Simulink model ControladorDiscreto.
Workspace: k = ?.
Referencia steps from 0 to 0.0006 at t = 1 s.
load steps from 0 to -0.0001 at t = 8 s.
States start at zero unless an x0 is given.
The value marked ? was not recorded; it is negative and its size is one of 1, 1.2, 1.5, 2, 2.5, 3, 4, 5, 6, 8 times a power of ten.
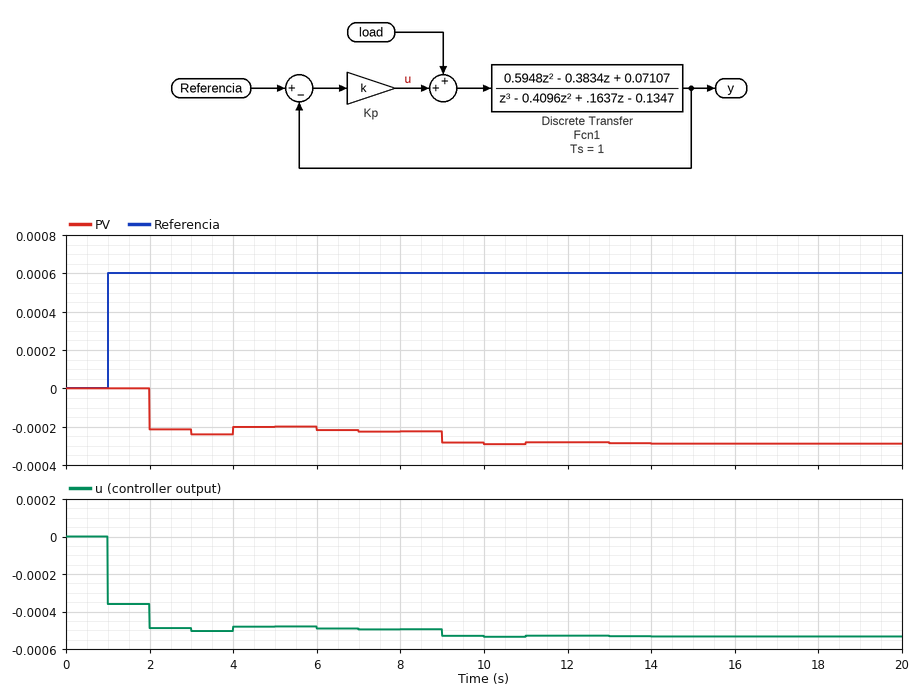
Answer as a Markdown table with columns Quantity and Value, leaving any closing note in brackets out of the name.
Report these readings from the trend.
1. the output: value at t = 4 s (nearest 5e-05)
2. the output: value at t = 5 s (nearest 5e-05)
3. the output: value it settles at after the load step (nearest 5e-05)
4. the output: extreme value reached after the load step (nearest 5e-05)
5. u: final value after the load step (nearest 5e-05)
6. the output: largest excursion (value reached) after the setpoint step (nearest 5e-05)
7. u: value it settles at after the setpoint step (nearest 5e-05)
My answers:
| Quantity | Value |
|---|---|
| the output: value at t = 4 s | -0.00020 |
| the output: value at t = 5 s | -0.00020 |
| the output: value it settles at after the load step | -0.00030 |
| the output: extreme value reached after the load step | -0.00030 |
| u: final value after the load step | -0.00055 |
| the output: largest excursion (value reached) after the setpoint step | -0.00025 |
| u: value it settles at after the setpoint step | -0.00050 |
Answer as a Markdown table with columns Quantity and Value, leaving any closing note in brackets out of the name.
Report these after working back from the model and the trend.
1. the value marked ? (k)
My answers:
| Quantity | Value |
|---|---|
| the value marked ? | -0.6 |
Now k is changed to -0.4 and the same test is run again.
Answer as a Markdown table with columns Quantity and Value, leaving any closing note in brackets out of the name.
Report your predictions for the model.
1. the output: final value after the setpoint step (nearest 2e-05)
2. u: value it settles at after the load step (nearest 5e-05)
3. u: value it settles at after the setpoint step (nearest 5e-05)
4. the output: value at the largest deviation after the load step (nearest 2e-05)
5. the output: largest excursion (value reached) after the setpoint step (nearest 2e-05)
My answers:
| Quantity | Value |
|---|---|
| the output: final value after the setpoint step | -0.00014 |
| u: value it settles at after the load step | -0.00030 |
| u: value it settles at after the setpoint step | -0.00030 |
| the output: value at the largest deviation after the load step | -0.00020 |
| the output: largest excursion (value reached) after the setpoint step | -0.00014 |
